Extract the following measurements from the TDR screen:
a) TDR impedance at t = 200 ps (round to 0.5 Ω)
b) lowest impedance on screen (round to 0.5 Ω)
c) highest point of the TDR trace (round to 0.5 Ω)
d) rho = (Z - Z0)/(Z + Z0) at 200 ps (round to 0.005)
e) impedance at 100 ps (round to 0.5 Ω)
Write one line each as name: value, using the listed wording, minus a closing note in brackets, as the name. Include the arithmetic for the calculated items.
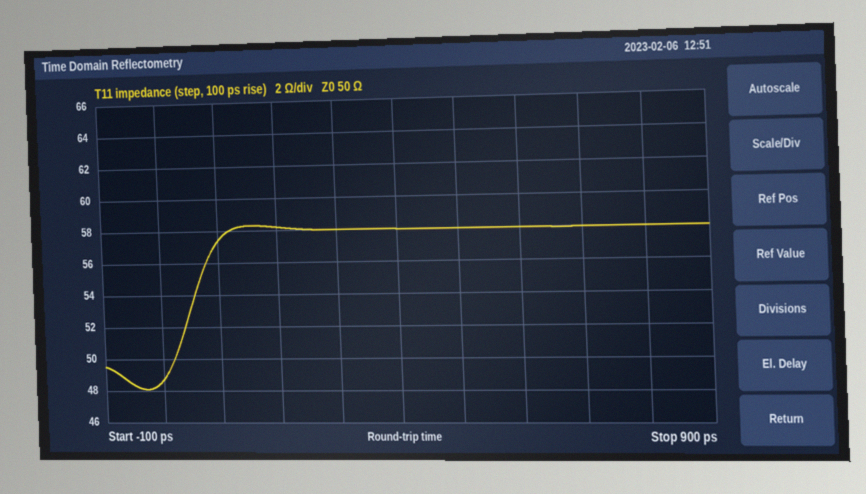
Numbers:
TDR impedance at t = 200 ps: 58.0 Ω
lowest impedance on screen: 48.0 Ω
highest point of the TDR trace: 58.5 Ω
rho = (Z - Z0)/(Z + Z0) at 200 ps: (58 − 50)/(58 + 50) ≈ +0.0741, so +0.075 to the nearest 0.005
impedance at 100 ps: 57.5 Ω
